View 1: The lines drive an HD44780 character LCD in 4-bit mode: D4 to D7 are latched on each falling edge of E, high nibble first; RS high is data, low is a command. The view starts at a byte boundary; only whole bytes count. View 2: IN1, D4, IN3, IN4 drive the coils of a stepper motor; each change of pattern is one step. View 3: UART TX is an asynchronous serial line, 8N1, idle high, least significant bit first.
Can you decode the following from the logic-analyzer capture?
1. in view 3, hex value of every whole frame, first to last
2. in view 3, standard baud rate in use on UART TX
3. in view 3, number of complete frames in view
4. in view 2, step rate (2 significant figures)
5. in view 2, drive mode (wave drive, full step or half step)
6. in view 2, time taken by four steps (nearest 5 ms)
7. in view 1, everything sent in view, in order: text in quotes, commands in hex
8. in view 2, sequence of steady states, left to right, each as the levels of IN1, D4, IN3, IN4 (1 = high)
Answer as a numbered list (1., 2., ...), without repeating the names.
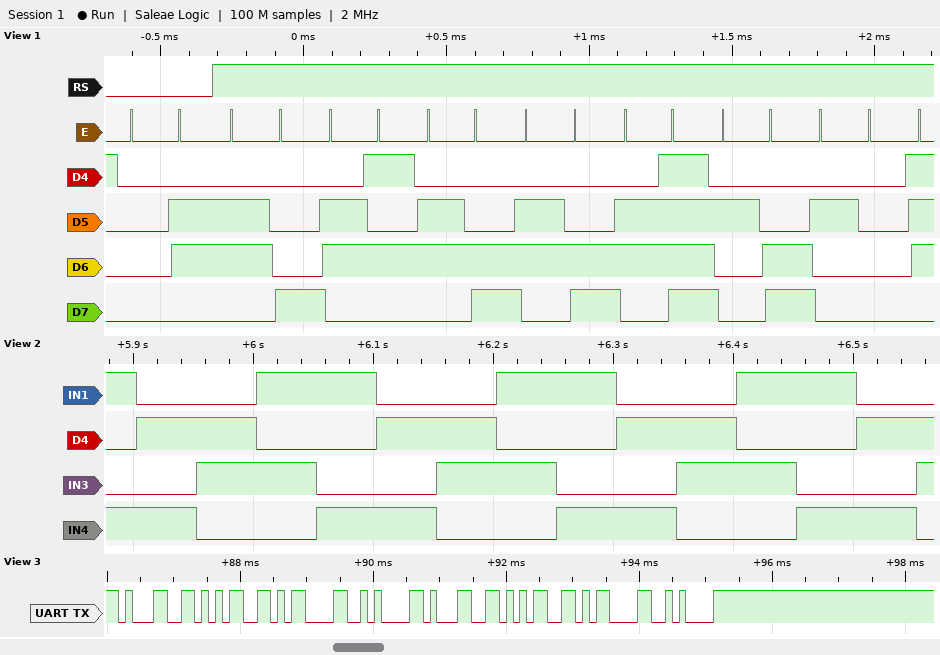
1. 31 35 0D 0A 31 35 0D 0A
2. 9600 baud
3. 8
4. 20 steps/s
5. full step
6. 200 ms
7. 0x06 "hello, "
8. 1001 0101 0110 1010 1001 0101 0110 1010 1001 0101 0110 1010 1001 0101 0110
